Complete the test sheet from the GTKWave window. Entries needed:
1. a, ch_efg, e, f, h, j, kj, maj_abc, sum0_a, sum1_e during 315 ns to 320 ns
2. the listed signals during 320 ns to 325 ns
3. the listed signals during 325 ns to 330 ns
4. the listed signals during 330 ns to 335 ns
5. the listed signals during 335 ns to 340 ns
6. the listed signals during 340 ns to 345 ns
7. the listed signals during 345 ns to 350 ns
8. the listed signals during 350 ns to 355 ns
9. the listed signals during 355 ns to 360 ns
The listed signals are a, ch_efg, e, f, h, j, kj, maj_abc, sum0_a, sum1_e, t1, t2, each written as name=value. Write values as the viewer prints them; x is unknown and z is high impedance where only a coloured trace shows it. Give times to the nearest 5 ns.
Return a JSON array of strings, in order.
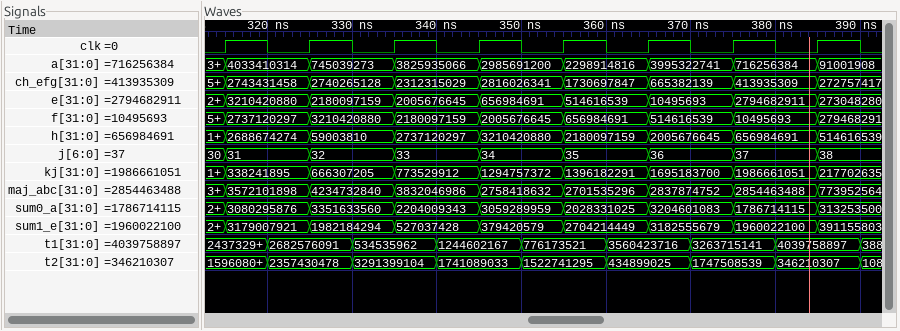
["a=4033410314, ch_efg=2743431458, e=3210420880, f=2737120297, h=2688674274, j=31, kj=338241895, maj_abc=3572101898, sum0_a=3080295876, sum1_e=3179007921", "a=4033410314, ch_efg=2743431458, e=3210420880, f=2737120297, h=2688674274, j=31, kj=338241895, maj_abc=3572101898, sum0_a=3080295876, sum1_e=3179007921, t1=2682576091, t2=2357430478", "a=745039273, ch_efg=2740265128, e=2180097159, f=3210420880, h=59003810, j=32, kj=666307205, maj_abc=4234732840, sum0_a=3351633560, sum1_e=1982184294, t1=2682576091, t2=2357430478", "a=745039273, ch_efg=2740265128, e=2180097159, f=3210420880, h=59003810, j=32, kj=666307205, maj_abc=4234732840, sum0_a=3351633560, sum1_e=1982184294, t1=534535962, t2=3291399104", "a=3825935066, ch_efg=2312315029, e=2005676645, f=2180097159, h=2737120297, j=33, kj=773529912, maj_abc=3832046986, sum0_a=2204009343, sum1_e=527037428, t1=534535962, t2=3291399104", "a=3825935066, ch_efg=2312315029, e=2005676645, f=2180097159, h=2737120297, j=33, kj=773529912, maj_abc=3832046986, sum0_a=2204009343, sum1_e=527037428, t1=1244602167, t2=1741089033", "a=2985691200, ch_efg=2816026341, e=656984691, f=2005676645, h=3210420880, j=34, kj=1294757372, maj_abc=2758418632, sum0_a=3059289959, sum1_e=379420579, t1=1244602167, t2=1741089033", "a=2985691200, ch_efg=2816026341, e=656984691, f=2005676645, h=3210420880, j=34, kj=1294757372, maj_abc=2758418632, sum0_a=3059289959, sum1_e=379420579, t1=776173521, t2=1522741295", "a=2298914816, ch_efg=1730697847, e=514616539, f=656984691, h=2180097159, j=35, kj=1396182291, maj_abc=2701535296, sum0_a=2028331025, sum1_e=2704214449, t1=776173521, t2=1522741295"]
